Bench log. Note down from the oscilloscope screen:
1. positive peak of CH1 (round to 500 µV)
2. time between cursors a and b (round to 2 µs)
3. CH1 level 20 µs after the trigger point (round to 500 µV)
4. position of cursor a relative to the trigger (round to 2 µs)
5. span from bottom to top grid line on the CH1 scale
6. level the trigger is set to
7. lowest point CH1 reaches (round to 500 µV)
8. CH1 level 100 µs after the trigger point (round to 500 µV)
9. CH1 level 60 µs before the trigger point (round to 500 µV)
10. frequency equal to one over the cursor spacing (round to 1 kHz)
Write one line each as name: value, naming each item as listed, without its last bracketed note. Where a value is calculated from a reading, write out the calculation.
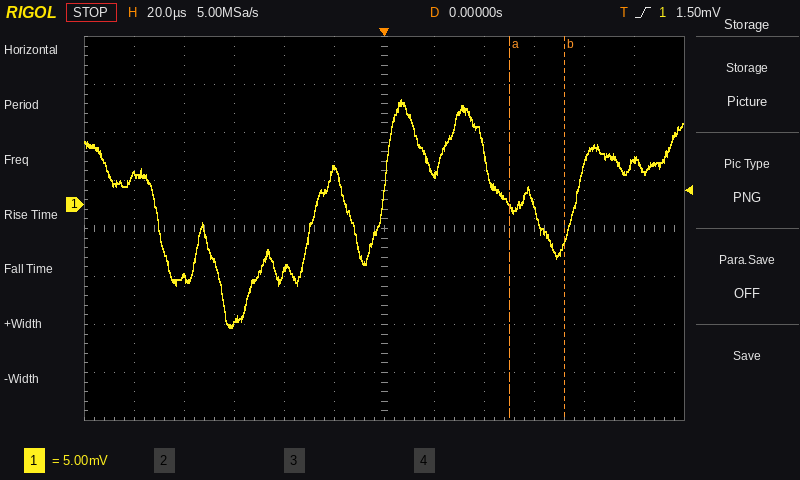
positive peak of CH1: 11.0 mV
time between cursors a and b: 22 µs
CH1 level 20 µs after the trigger point: 3.0 mV
position of cursor a relative to the trigger: +50 µs
span from bottom to top grid line on the CH1 scale: 40 mV
level the trigger is set to: 1.50 mV
lowest point CH1 reaches: -13.0 mV
CH1 level 100 µs after the trigger point: 4.5 mV
CH1 level 60 µs before the trigger point: -12.5 mV
frequency equal to one over the cursor spacing: 1 / 22 µs ≈ 45 kHz
